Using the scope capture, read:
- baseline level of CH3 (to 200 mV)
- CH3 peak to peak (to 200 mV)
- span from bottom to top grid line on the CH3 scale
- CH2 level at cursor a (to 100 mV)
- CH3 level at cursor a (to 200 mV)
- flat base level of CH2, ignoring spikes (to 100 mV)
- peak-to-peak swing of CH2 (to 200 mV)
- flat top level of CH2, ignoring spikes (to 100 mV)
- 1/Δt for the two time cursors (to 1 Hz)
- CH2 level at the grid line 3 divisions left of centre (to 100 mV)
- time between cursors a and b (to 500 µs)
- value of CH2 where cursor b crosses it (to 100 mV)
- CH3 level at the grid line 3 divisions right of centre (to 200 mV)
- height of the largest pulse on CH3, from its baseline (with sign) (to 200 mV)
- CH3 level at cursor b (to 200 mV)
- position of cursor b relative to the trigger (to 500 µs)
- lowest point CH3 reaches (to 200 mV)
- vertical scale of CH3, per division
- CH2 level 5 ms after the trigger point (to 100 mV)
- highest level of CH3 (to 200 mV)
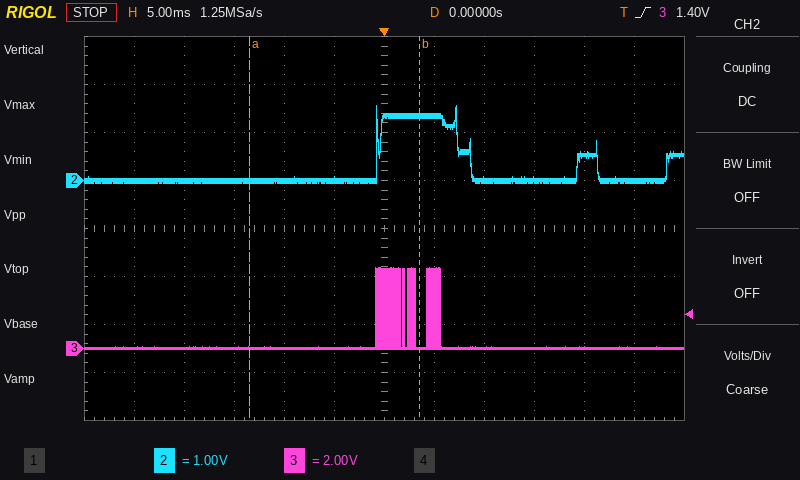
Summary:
0.0 V
3.4 V
16 V
0.0 V
0.0 V
0.0 V
1.6 V
1.4 V
59 Hz
0.0 V
17.0 ms
1.4 V
0.0 V
+3.4 V
0.0 V
+3.5 ms
0.0 V
2 V
1.4 V
3.4 V
